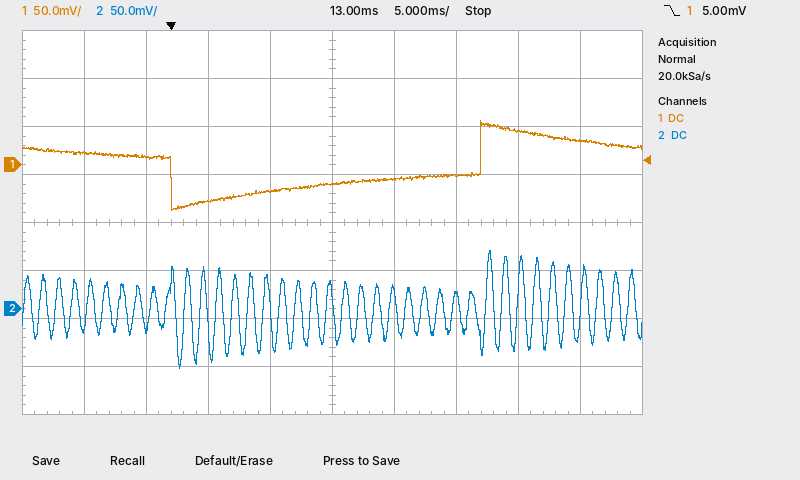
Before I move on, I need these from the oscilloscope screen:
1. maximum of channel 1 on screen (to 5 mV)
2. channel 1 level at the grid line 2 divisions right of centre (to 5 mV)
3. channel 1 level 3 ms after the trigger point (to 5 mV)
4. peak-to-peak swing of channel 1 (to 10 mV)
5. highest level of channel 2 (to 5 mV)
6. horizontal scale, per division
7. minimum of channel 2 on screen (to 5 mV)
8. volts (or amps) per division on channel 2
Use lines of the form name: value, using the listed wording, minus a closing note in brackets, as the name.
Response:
maximum of channel 1 on screen: 45 mV
channel 1 level at the grid line 2 divisions right of centre: -10 mV
channel 1 level 3 ms after the trigger point: -40 mV
peak-to-peak swing of channel 1: 90 mV
highest level of channel 2: 60 mV
horizontal scale, per division: 5 ms
minimum of channel 2 on screen: -60 mV
volts (or amps) per division on channel 2: 50 mV
